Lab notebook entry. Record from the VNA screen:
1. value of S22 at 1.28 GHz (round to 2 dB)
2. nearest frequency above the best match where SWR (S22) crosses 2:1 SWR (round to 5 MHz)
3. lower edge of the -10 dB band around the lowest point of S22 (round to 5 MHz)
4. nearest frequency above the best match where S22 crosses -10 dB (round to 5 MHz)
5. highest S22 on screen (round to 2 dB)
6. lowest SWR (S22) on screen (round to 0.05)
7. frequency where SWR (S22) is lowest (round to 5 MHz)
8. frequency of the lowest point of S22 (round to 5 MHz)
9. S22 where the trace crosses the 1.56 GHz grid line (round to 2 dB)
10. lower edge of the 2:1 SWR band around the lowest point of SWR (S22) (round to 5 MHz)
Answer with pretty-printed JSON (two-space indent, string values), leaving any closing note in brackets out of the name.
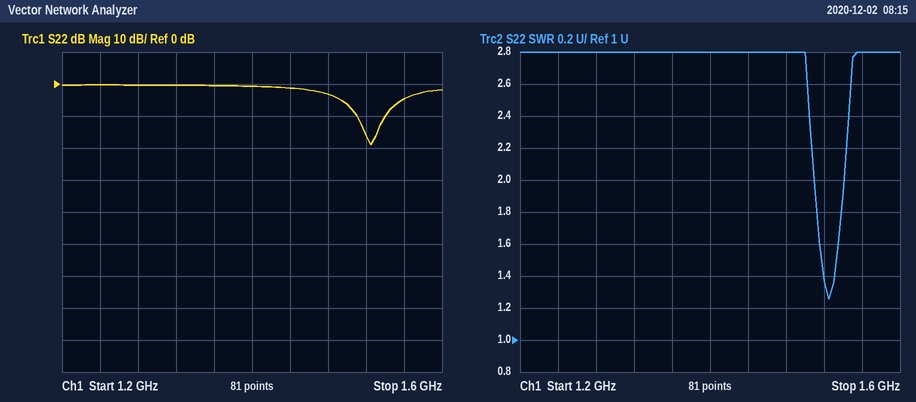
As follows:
{
  "value of S22 at 1.28 GHz": "0 dB",
  "nearest frequency above the best match where SWR (S22) crosses 2:1 SWR": "1.540 GHz",
  "lower edge of the -10 dB band around the lowest point of S22": "1.510 GHz",
  "nearest frequency above the best match where S22 crosses -10 dB": "1.540 GHz",
  "highest S22 on screen": "0 dB",
  "lowest SWR (S22) on screen": "1.25",
  "frequency where SWR (S22) is lowest": "1.525 GHz",
  "frequency of the lowest point of S22": "1.525 GHz",
  "S22 where the trace crosses the 1.56 GHz grid line": "-4 dB",
  "lower edge of the 2:1 SWR band around the lowest point of SWR (S22)": "1.510 GHz"
}
